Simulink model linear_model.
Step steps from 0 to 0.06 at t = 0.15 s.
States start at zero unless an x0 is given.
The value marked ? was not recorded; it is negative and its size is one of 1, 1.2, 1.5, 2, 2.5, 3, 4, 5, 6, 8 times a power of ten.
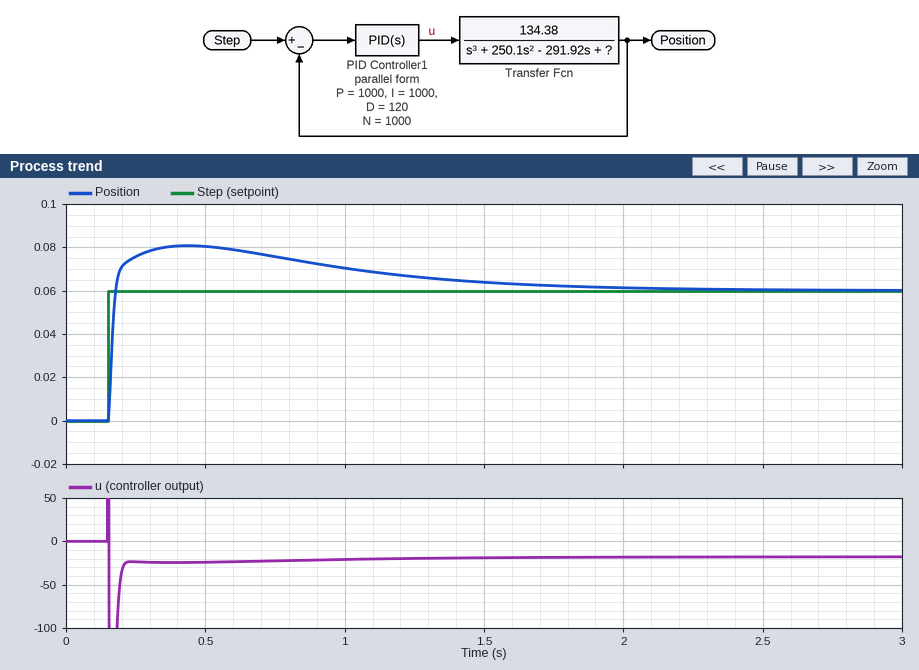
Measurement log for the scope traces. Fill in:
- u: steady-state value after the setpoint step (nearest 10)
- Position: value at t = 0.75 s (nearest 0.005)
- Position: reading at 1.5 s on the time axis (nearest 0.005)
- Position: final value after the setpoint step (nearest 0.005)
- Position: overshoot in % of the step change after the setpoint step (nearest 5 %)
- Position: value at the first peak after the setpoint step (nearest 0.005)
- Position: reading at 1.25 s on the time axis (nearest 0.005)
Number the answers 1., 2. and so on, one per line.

1. -20
2. 0.075
3. 0.065
4. 0.060
5. 35 %
6. 0.080
7. 0.065
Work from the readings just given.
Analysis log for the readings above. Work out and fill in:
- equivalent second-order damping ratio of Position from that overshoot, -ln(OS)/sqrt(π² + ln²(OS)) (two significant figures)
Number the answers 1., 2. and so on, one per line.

1. 0.32
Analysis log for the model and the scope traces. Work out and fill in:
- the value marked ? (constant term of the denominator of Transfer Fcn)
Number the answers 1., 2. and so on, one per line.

1. -40000
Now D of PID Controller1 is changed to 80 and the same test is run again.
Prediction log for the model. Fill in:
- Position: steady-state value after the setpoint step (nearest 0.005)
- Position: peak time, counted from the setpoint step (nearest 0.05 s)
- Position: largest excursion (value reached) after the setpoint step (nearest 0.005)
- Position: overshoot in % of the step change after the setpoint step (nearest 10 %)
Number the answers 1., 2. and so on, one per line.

1. 0.060
2. 0.15 s
3. 0.085
4. 40 %
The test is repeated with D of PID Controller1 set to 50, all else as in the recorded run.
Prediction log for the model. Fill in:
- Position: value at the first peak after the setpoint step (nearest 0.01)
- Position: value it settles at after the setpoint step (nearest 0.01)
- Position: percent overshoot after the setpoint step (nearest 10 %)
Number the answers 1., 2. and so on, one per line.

1. 0.10
2. 0.06
3. 70 %
